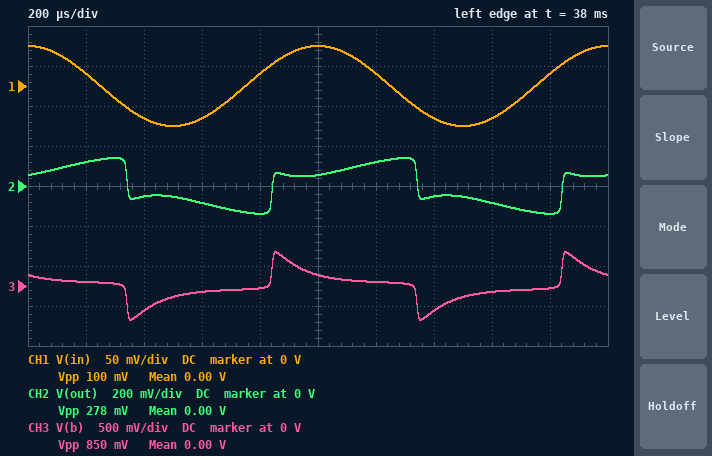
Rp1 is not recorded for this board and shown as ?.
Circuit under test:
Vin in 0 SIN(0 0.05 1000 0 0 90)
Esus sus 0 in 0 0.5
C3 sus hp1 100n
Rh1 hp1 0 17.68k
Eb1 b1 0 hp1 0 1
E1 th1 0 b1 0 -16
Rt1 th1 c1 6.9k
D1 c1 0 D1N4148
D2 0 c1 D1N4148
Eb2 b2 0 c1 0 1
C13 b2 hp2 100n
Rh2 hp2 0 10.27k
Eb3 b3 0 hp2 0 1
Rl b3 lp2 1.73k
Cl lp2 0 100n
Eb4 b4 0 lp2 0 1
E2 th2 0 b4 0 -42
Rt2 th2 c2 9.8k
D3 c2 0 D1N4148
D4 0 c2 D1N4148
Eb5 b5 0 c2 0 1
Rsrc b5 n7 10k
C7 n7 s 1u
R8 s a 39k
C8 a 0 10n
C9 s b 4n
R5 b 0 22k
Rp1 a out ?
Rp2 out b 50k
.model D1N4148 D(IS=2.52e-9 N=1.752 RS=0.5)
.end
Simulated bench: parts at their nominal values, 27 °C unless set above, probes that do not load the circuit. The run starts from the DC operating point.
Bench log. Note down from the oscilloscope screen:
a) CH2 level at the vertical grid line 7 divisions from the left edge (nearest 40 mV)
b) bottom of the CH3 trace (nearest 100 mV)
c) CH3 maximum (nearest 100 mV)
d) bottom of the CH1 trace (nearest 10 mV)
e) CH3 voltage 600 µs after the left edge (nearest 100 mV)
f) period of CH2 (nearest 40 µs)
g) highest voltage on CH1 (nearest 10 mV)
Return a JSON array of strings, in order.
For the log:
["-40 mV", "-400 mV", "400 mV", "-50 mV", "-100 mV", "1.00 ms", "50 mV"]
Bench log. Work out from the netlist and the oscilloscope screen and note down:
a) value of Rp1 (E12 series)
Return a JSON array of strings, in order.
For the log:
["39 kΩ"]
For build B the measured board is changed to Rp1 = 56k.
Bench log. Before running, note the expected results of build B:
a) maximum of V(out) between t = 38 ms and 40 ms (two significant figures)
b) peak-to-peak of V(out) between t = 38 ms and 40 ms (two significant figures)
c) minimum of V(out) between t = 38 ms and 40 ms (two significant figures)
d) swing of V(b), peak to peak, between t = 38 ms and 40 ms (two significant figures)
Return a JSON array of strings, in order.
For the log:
["130 mV", "250 mV", "-130 mV", "870 mV"]
